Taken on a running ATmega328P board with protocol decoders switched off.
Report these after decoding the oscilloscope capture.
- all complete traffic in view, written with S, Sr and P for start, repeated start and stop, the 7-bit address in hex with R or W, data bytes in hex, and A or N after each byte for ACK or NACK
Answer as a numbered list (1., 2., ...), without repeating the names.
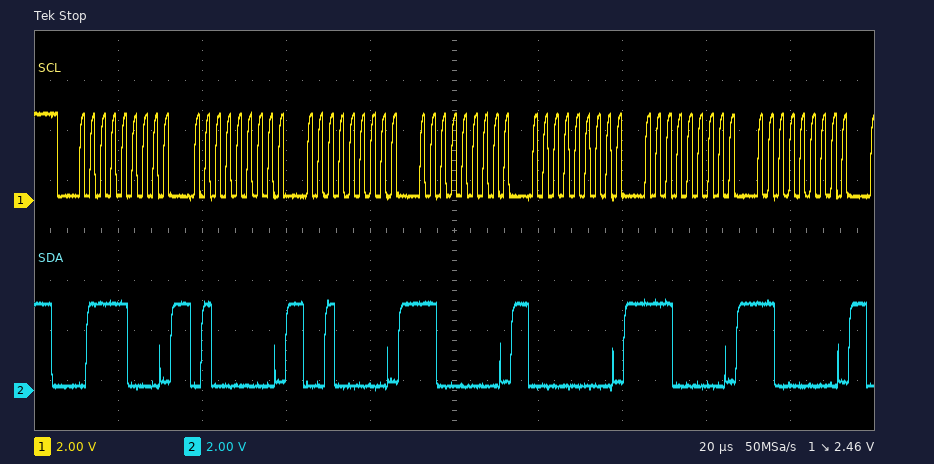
1. S 3CW A 40 A 20 A C0 A 00 A E0 A C0 A
